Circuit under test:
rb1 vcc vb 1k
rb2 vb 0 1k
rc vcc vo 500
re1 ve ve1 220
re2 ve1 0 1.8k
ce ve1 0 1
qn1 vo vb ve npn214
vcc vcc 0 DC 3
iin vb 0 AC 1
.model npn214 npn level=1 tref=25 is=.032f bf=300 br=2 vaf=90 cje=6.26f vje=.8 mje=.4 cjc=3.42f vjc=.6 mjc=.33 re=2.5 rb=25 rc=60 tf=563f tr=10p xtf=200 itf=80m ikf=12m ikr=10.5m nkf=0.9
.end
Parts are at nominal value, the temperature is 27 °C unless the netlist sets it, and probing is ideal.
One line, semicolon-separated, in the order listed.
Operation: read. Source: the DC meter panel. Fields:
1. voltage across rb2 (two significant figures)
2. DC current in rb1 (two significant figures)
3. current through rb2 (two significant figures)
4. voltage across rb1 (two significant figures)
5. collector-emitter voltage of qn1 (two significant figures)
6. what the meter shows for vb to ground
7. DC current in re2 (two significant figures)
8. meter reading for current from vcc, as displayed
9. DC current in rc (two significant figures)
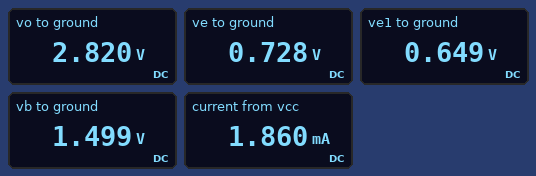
1.5 V; 1.5 mA; 1.5 mA; 1.5 V; 2.1 V; 1.499 V; 360 µA; 1.860 mA; 360 µA
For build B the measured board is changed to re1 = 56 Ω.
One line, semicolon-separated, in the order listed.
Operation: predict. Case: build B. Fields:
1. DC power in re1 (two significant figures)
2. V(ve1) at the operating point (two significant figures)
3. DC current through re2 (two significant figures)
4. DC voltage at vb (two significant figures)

8.6 µW; 700 mV; 390 µA; 1.5 V
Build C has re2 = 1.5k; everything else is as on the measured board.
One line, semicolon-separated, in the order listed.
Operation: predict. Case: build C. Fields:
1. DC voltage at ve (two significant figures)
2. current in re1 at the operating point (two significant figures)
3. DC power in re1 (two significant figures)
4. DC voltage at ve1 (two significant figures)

720 mV; 420 µA; 39 µW; 630 mV
